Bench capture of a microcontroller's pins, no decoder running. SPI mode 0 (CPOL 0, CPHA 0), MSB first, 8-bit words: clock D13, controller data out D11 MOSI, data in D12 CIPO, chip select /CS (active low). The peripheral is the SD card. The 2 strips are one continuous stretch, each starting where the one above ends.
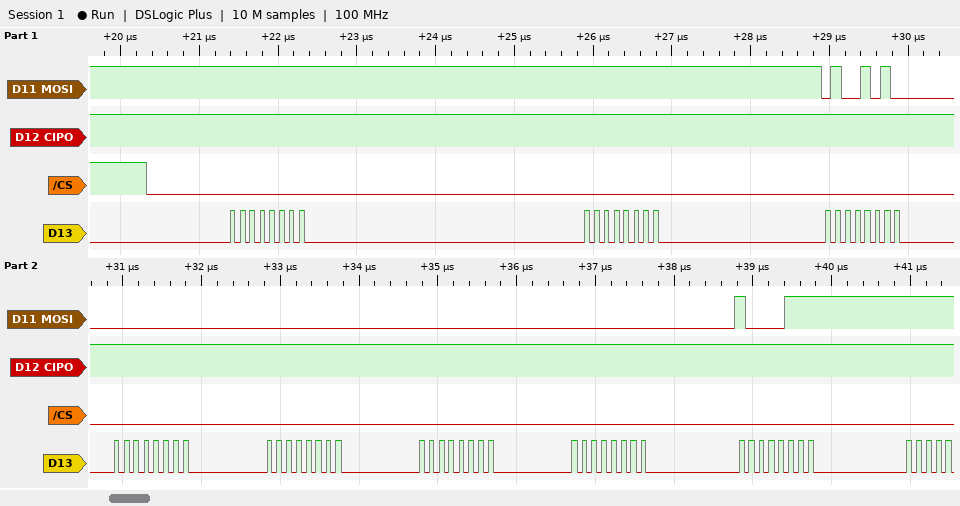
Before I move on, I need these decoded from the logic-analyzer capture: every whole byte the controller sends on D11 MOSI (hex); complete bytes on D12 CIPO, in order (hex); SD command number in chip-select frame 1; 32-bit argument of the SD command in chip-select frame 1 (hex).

FF FF 4A 00 00 00 00 87
FF FF FF FF FF FF FF FF
CMD10
0x00000000
